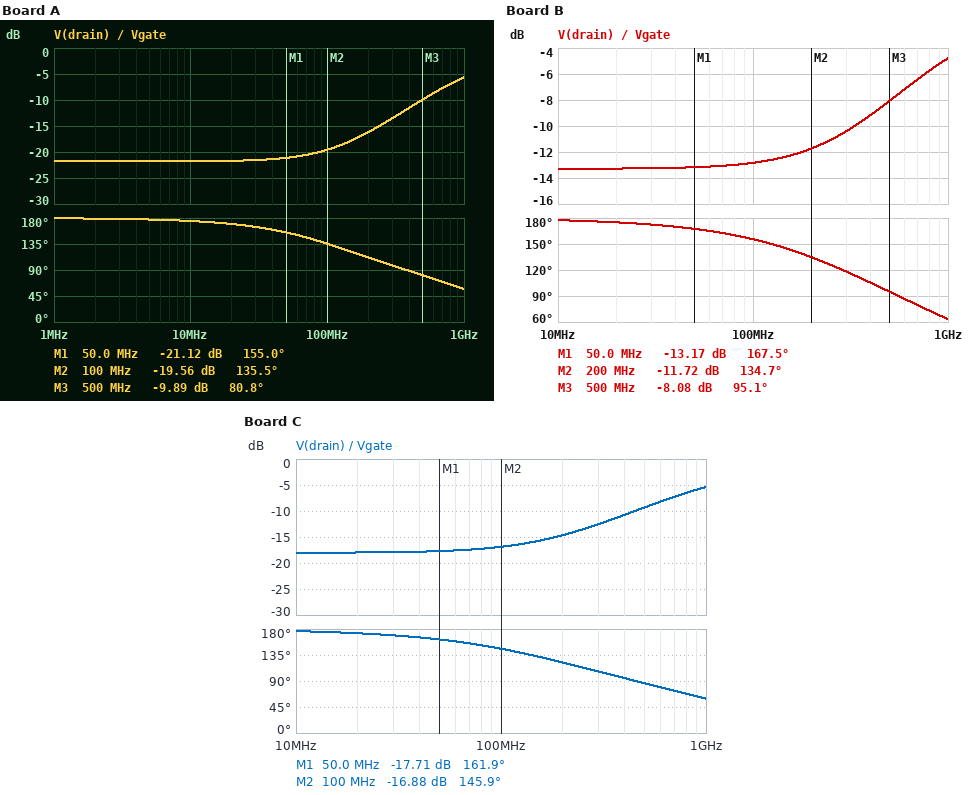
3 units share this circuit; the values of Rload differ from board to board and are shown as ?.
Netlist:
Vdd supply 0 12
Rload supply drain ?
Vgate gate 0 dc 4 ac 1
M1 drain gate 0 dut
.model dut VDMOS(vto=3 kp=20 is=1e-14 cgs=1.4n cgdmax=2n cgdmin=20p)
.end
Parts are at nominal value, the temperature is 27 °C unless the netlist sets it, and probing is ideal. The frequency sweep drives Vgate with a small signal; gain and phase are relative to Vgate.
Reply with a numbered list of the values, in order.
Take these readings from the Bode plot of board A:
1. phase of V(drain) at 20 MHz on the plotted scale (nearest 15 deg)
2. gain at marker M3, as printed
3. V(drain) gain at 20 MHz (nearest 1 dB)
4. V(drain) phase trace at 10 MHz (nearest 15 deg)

1. 165 deg
2. -9.89 dB
3. -22 dB
4. 180 deg
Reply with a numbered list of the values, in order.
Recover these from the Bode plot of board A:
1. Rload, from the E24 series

1. 8.2 Ω
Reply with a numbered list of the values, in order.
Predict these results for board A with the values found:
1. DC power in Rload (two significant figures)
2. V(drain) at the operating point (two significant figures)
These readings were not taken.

1. 17 W
2. 76 mV
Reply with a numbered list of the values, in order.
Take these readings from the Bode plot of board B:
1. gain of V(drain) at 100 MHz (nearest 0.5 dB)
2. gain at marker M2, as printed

1. -13.0 dB
2. -11.72 dB
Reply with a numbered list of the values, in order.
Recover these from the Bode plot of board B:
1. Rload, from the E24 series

1. 3.6 Ω
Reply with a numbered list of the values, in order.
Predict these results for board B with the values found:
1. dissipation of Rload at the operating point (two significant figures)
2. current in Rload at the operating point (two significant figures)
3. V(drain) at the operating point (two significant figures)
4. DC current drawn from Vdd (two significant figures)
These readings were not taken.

1. 39 W
2. 3.3 A
3. 180 mV
4. 3.3 A
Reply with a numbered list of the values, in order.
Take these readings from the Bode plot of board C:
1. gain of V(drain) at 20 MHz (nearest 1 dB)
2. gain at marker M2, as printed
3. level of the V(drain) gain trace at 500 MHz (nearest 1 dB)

1. -18 dB
2. -16.88 dB
3. -9 dB
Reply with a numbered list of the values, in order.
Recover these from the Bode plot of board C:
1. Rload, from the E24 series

1. 5.6 Ω
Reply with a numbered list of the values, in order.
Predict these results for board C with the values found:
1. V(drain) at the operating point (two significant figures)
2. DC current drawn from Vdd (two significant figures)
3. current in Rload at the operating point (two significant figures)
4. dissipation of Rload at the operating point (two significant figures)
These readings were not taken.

1. 110 mV
2. 2.1 A
3. 2.1 A
4. 25 W
